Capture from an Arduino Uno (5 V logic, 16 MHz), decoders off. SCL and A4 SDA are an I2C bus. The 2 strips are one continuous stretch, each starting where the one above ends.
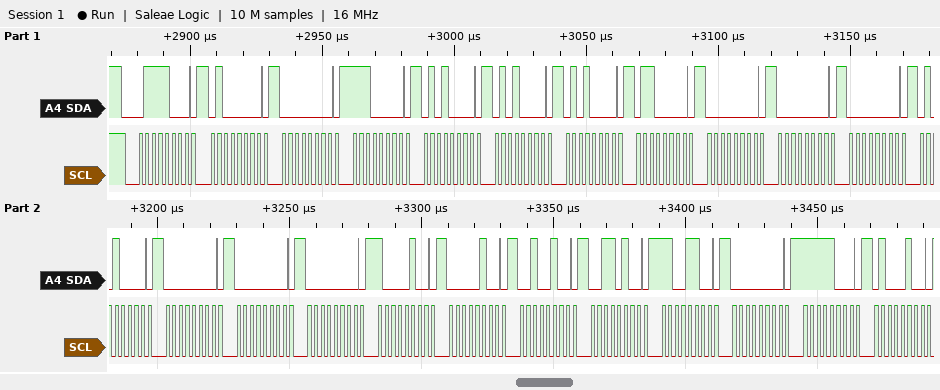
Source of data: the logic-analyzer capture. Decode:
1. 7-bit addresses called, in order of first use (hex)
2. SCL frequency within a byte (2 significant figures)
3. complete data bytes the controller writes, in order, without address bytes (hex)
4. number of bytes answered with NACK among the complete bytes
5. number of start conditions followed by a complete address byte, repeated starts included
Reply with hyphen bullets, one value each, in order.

- 0x3C
- 400 kHz
- 40 00 E0 50 50 50 60 00 00 00 50 00 00 00 84 04 24 34 CC 00 F8 44
- 0
- 1
